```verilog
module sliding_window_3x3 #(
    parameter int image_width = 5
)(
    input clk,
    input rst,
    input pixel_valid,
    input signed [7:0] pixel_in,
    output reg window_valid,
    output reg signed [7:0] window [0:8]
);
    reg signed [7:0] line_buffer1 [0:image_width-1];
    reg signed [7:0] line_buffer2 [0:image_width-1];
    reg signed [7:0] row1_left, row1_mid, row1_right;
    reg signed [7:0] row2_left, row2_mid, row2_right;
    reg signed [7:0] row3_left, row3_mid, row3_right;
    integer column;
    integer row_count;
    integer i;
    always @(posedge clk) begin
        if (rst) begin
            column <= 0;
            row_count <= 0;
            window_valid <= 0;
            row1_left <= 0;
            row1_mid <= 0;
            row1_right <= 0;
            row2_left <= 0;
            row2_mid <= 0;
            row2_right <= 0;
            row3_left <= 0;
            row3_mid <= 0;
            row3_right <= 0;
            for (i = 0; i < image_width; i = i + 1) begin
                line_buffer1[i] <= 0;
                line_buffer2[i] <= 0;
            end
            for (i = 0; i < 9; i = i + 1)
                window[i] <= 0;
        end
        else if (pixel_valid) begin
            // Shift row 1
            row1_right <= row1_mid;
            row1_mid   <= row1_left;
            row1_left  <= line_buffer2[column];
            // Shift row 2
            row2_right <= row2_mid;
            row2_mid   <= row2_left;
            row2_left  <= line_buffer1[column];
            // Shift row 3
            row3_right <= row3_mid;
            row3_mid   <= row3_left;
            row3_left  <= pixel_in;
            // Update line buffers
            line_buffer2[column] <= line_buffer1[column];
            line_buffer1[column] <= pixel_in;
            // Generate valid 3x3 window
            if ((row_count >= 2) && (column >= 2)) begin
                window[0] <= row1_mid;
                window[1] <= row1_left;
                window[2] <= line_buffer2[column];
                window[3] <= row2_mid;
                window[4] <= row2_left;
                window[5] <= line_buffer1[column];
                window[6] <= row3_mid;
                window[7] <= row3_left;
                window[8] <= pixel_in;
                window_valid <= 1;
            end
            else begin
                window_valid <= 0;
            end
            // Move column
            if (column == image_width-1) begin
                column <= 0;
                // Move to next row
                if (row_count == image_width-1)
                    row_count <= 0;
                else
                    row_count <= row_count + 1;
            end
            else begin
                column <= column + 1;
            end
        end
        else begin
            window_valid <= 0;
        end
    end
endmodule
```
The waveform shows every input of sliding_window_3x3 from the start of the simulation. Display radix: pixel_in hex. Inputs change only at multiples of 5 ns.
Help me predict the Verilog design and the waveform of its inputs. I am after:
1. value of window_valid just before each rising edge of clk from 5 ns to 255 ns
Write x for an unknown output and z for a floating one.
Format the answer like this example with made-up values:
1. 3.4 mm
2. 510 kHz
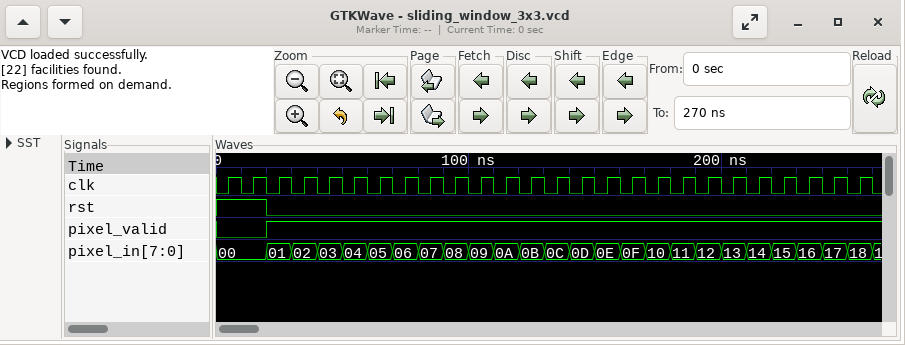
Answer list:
1. x 0 0 0 0 0 0 0 0 0 0 0 0 0 0 1 1 1 0 0 1 1 1 0 0 1
